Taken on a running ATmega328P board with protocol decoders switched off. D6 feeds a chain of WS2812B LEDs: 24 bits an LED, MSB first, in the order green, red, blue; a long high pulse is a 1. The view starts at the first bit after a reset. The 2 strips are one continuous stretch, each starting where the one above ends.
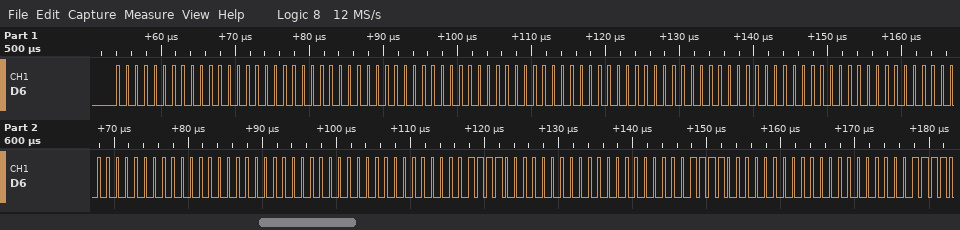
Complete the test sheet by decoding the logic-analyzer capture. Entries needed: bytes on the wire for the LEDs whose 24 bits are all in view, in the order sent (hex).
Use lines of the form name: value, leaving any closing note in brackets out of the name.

bytes on the wire for the LEDs whose 24 bits are all in view, in the order sent: 00 00 00 00 00 00 00 00 00 00 00 00 00 00 00 00 1E 00 00 1E 00
